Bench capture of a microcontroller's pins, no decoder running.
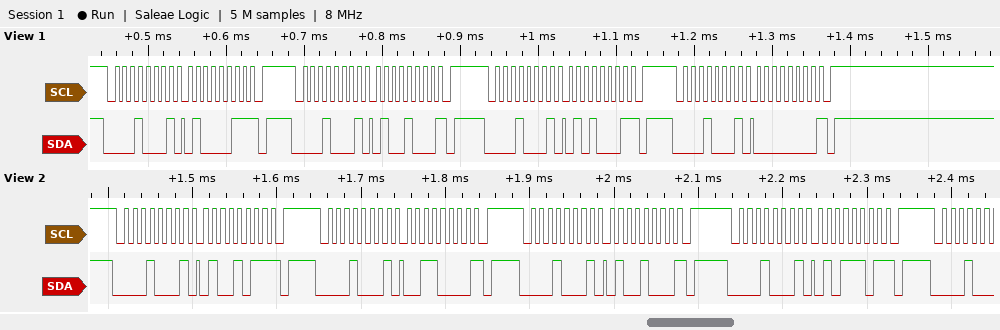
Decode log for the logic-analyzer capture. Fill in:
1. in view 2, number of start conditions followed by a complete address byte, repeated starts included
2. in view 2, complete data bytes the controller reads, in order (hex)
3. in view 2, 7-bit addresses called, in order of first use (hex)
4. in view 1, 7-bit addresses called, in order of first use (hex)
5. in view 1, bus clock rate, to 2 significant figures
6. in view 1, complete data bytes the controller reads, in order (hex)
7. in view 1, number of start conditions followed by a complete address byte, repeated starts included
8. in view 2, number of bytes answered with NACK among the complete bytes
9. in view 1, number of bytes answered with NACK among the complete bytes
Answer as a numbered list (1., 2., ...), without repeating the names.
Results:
1. 4
2. 4B 30 48 5D
3. 0x08
4. 0x08
5. 100 kHz
6. 43 48 51 00
7. 4
8. 4
9. 4
